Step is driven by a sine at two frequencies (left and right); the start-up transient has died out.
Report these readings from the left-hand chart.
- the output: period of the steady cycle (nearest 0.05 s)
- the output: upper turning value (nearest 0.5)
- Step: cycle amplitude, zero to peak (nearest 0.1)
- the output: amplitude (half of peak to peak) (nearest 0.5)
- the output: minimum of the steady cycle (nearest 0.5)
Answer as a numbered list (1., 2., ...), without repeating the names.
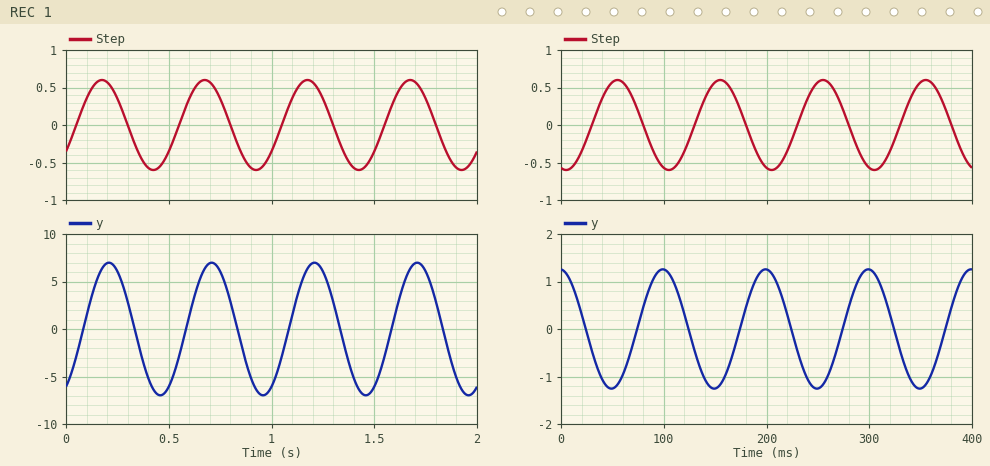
1. 0.50 s
2. 7.0
3. 0.6
4. 7.0
5. -7.0
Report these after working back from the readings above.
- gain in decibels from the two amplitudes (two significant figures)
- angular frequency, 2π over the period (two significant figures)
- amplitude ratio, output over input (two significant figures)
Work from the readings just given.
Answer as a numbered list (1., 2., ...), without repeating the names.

1. 21 dB
2. 13 rad/s
3. 12
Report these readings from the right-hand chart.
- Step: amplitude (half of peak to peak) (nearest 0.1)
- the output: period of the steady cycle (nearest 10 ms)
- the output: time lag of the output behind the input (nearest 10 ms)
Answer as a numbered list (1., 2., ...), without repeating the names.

1. 0.6
2. 100 ms
3. 40 ms
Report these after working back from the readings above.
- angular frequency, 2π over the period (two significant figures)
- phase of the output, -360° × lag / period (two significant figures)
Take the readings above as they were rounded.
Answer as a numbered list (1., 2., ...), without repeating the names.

1. 0.063 rad/ms
2. -140°
